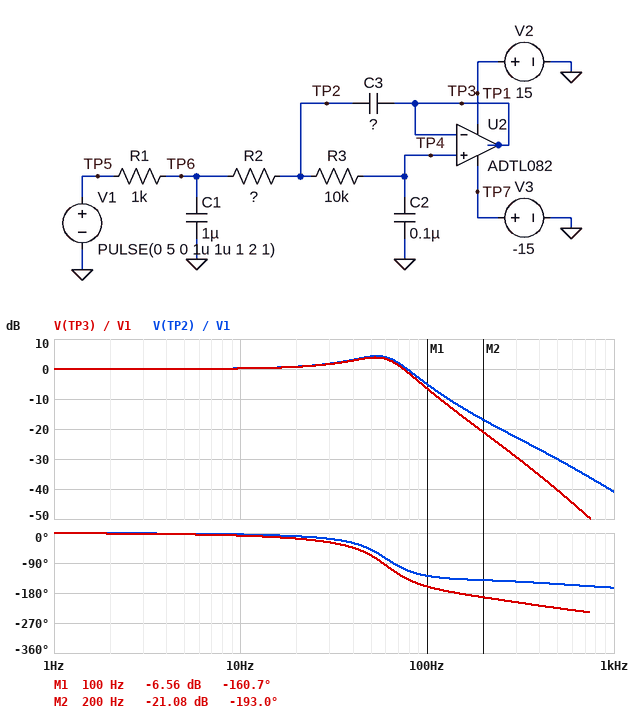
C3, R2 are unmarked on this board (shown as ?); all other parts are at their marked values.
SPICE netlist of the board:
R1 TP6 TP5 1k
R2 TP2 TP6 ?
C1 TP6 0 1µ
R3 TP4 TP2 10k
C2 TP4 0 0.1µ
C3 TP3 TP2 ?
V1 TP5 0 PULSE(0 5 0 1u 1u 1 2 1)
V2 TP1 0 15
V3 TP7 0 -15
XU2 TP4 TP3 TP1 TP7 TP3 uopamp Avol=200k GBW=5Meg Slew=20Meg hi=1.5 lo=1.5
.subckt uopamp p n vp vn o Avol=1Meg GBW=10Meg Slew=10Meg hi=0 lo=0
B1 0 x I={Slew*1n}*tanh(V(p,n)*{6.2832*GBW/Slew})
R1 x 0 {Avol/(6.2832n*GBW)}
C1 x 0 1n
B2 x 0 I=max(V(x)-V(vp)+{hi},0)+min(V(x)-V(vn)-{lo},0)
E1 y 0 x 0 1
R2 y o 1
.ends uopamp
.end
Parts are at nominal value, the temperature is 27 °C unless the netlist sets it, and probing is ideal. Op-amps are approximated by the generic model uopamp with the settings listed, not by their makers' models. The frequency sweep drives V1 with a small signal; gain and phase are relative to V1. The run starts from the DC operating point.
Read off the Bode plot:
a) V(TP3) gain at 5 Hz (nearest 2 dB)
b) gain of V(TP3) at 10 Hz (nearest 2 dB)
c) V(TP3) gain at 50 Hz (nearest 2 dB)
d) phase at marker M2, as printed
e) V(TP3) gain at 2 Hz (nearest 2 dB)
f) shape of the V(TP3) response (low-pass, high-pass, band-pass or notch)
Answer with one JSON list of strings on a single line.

["0 dB", "0 dB", "4 dB", "-193.0 deg", "0 dB", "low-pass"]
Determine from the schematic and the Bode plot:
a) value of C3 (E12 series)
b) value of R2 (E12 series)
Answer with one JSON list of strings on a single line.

["3.9 µF", "680 Ω"]
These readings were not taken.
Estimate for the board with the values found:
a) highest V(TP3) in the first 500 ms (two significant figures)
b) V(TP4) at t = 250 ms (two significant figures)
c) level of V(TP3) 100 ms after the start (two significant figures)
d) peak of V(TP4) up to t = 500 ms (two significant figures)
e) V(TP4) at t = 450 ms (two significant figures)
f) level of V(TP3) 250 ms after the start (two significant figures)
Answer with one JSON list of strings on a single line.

["6.6 V", "5.0 V", "5.0 V", "6.6 V", "5.0 V", "5.0 V"]
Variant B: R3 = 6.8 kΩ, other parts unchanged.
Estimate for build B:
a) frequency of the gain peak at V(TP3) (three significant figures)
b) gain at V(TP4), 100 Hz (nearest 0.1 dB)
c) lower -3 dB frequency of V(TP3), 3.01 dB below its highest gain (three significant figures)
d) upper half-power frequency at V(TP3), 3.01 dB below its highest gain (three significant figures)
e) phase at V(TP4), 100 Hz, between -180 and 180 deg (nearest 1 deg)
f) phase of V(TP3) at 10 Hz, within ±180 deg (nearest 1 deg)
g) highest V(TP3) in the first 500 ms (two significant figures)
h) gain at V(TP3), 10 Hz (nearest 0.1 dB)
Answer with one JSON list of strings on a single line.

["64.6 Hz", "-2.1 dB", "25.6 Hz", "87.3 Hz", "-146 deg", "-7 deg", "6.6 V", "0.1 dB"]
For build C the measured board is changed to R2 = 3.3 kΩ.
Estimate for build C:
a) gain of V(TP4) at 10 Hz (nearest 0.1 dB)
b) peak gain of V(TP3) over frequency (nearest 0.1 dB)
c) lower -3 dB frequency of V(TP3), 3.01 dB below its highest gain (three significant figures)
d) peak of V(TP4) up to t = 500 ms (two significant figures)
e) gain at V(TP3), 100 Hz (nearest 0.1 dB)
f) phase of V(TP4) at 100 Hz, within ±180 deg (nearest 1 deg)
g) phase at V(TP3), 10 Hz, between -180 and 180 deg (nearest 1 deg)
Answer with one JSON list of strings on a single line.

["0.5 dB", "7.9 dB", "27.8 Hz", "7.6 V", "-16.1 dB", "165 deg", "-9 deg"]
